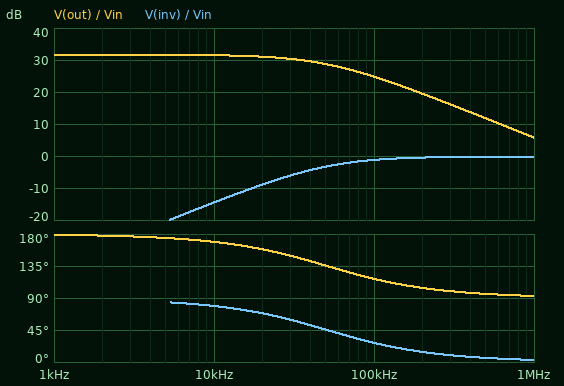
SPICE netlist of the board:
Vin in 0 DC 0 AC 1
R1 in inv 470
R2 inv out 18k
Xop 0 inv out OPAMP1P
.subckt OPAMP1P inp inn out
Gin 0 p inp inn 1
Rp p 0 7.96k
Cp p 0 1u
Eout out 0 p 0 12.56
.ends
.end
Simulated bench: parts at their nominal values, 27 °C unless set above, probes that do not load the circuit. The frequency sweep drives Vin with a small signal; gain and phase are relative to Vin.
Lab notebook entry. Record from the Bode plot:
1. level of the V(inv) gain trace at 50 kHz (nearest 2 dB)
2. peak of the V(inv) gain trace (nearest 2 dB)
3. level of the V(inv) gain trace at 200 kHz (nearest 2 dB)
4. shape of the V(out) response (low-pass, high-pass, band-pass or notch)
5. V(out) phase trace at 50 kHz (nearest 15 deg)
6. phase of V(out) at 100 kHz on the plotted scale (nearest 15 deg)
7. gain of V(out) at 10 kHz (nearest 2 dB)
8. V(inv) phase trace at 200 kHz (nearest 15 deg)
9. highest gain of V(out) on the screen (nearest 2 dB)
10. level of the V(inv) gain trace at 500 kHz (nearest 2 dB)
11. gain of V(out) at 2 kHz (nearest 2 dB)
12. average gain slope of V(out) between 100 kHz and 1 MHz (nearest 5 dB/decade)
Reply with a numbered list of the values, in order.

1. -4 dB
2. 0 dB
3. 0 dB
4. low-pass
5. 135 deg
6. 120 deg
7. 32 dB
8. 15 deg
9. 32 dB
10. 0 dB
11. 32 dB
12. -20 dB/decade
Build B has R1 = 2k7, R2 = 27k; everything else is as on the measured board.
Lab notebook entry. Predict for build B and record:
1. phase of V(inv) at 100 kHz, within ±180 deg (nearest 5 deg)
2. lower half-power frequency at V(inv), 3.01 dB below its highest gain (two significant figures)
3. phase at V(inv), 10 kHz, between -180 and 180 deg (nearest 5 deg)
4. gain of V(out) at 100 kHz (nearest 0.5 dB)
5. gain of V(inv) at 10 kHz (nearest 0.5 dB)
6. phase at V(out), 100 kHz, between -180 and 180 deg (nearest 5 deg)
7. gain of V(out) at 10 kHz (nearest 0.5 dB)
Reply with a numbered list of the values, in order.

1. 60 deg
2. 180 kHz
3. 85 deg
4. 19.0 dB
5. -26.0 dB
6. 150 deg
7. 20.0 dB
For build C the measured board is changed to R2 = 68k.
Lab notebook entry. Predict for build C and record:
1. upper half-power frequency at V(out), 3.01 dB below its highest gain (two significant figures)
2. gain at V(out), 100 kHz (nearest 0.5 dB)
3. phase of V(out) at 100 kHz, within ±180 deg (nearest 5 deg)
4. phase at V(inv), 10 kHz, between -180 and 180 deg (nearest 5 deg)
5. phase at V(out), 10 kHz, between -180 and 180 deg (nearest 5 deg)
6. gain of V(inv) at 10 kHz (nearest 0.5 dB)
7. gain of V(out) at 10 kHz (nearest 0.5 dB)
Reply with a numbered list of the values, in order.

1. 14 kHz
2. 26.0 dB
3. 100 deg
4. 55 deg
5. 145 deg
6. -4.5 dB
7. 41.5 dB
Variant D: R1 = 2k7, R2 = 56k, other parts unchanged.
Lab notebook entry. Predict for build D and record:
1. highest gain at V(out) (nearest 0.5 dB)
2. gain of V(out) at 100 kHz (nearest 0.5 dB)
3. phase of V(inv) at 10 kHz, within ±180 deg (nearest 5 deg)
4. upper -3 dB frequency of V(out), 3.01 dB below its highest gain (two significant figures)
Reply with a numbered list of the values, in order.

1. 26.5 dB
2. 23.0 dB
3. 85 deg
4. 92 kHz
